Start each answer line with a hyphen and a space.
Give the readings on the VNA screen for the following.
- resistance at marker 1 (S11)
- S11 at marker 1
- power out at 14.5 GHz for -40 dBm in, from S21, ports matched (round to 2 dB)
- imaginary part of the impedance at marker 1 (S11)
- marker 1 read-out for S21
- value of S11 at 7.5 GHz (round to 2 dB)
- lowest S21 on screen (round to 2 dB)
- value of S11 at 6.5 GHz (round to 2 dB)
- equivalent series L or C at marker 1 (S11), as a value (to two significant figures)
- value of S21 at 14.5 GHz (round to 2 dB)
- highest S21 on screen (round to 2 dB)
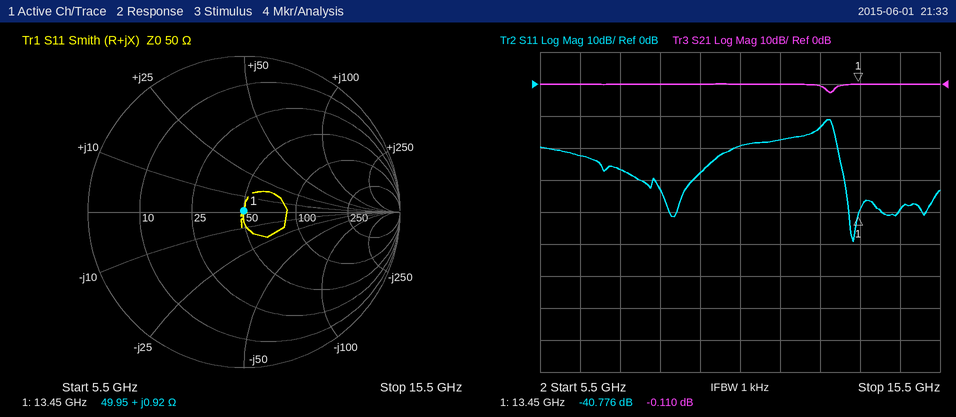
- 49.95 Ω
- -40.776 dB
- -40 dBm
- +0.92 Ω
- -0.110 dB
- -26 dB
- -2 dB
- -22 dB
- 11 pH
- 0 dB
- 0 dB
